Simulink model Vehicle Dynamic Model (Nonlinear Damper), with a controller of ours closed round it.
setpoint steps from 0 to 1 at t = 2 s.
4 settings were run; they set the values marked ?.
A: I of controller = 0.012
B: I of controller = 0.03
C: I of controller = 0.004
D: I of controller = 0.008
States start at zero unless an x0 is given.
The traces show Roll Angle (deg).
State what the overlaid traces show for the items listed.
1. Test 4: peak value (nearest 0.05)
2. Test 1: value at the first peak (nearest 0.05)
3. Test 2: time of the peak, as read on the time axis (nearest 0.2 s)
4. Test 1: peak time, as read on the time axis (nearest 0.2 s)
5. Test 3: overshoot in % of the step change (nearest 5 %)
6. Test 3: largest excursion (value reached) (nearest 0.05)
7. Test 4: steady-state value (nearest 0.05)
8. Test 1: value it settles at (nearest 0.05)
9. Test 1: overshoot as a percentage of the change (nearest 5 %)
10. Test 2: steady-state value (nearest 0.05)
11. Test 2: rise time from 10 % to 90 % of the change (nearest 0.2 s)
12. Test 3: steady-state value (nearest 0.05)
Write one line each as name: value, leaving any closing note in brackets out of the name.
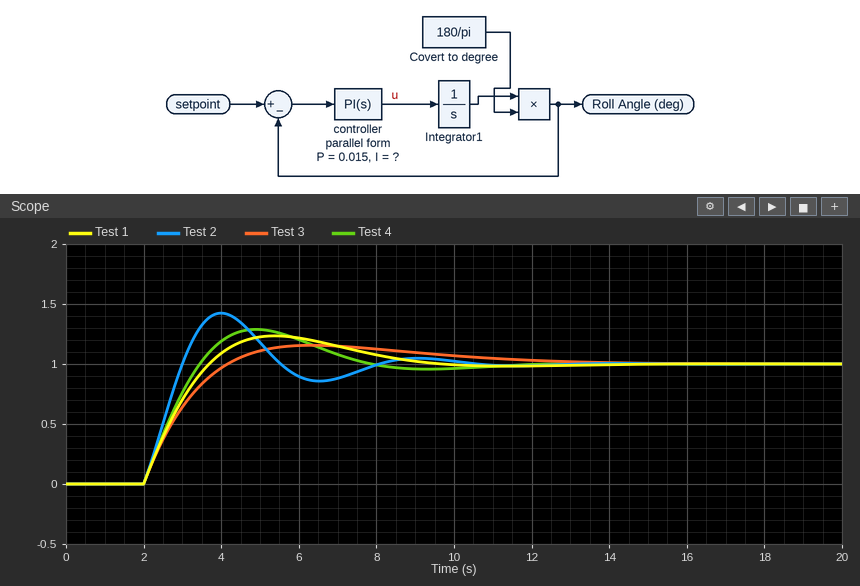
Test 4: peak value: 1.30
Test 1: value at the first peak: 1.25
Test 2: time of the peak, as read on the time axis: 4.0 s
Test 1: peak time, as read on the time axis: 5.4 s
Test 3: overshoot in % of the step change: 15 %
Test 3: largest excursion (value reached): 1.15
Test 4: steady-state value: 1.00
Test 1: value it settles at: 1.00
Test 1: overshoot as a percentage of the change: 25 %
Test 2: steady-state value: 1.00
Test 2: rise time from 10 % to 90 % of the change: 0.8 s
Test 3: steady-state value: 1.00
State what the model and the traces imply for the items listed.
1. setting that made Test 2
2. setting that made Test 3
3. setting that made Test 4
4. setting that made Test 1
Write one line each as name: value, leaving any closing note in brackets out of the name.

setting that made Test 2: B
setting that made Test 3: C
setting that made Test 4: A
setting that made Test 1: D
